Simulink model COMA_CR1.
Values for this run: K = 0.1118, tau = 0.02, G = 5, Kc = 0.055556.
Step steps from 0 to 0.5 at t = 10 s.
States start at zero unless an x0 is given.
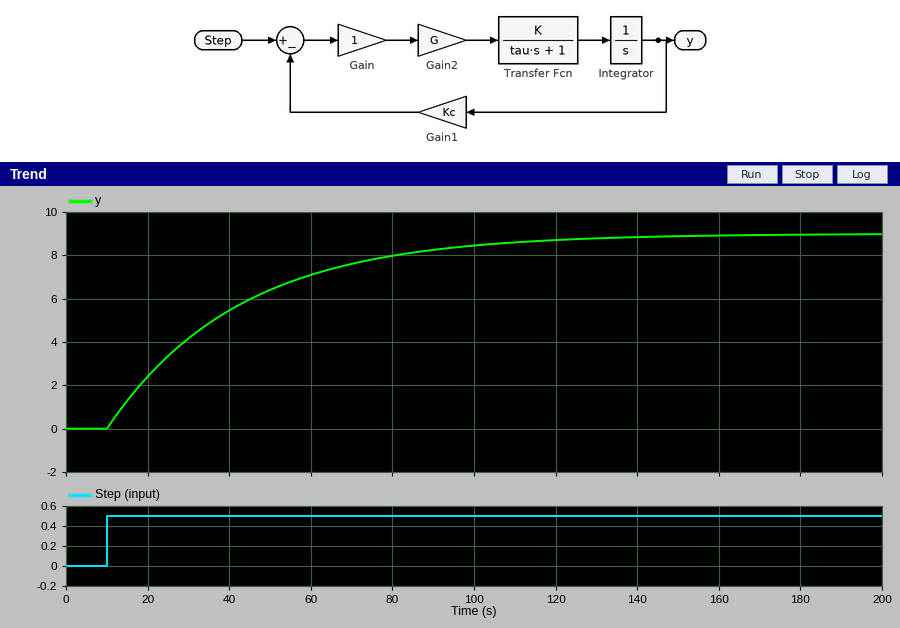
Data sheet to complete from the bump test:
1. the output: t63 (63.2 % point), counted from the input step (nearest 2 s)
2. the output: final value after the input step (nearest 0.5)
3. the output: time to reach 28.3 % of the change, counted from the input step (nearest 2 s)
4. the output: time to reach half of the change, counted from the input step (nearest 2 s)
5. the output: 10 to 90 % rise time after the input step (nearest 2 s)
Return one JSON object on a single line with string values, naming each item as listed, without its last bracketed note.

{"the output: t63 (63.2 % point), counted from the input step": "32 s", "the output: final value after the input step": "9.0", "the output: time to reach 28.3 % of the change, counted from the input step": "10 s", "the output: time to reach half of the change, counted from the input step": "22 s", "the output: 10 to 90 % rise time after the input step": "70 s"}
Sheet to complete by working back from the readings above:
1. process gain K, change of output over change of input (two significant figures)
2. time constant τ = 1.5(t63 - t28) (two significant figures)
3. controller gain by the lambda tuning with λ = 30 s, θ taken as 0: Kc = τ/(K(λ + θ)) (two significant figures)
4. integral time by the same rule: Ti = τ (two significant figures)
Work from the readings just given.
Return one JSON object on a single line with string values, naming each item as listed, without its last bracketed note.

{"process gain K, change of output over change of input": "18", "time constant τ = 1.5(t63 - t28)": "33 s", "controller gain by the lambda tuning with λ = 30 s, θ taken as 0: Kc = τ/(K(λ + θ))": "0.061", "integral time by the same rule: Ti = τ": "33 s"}
